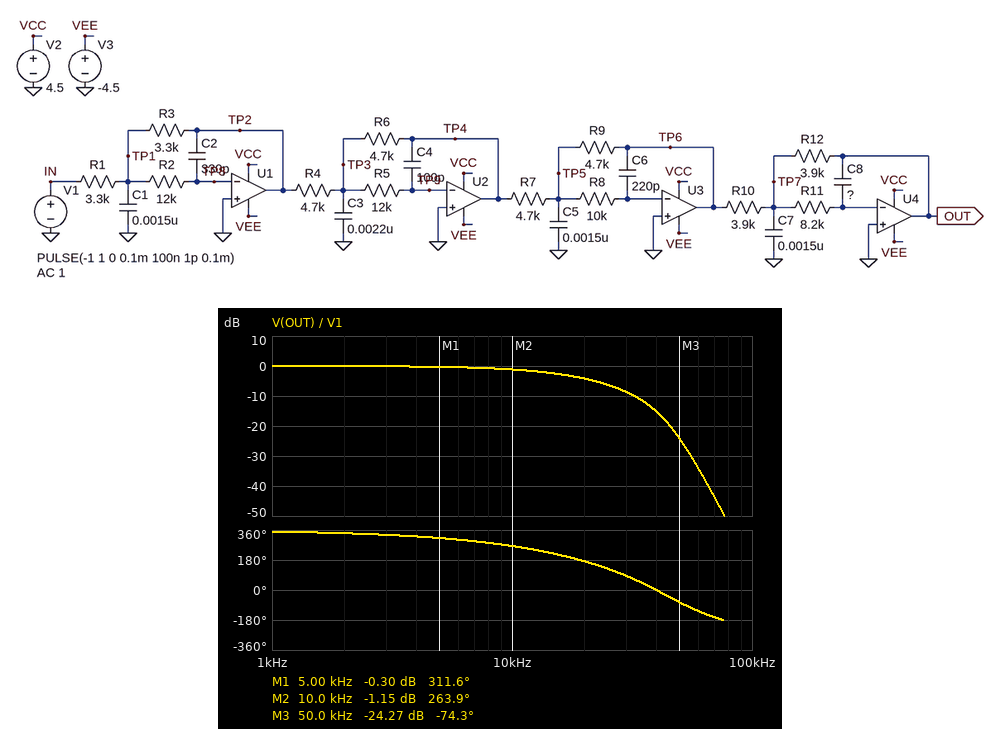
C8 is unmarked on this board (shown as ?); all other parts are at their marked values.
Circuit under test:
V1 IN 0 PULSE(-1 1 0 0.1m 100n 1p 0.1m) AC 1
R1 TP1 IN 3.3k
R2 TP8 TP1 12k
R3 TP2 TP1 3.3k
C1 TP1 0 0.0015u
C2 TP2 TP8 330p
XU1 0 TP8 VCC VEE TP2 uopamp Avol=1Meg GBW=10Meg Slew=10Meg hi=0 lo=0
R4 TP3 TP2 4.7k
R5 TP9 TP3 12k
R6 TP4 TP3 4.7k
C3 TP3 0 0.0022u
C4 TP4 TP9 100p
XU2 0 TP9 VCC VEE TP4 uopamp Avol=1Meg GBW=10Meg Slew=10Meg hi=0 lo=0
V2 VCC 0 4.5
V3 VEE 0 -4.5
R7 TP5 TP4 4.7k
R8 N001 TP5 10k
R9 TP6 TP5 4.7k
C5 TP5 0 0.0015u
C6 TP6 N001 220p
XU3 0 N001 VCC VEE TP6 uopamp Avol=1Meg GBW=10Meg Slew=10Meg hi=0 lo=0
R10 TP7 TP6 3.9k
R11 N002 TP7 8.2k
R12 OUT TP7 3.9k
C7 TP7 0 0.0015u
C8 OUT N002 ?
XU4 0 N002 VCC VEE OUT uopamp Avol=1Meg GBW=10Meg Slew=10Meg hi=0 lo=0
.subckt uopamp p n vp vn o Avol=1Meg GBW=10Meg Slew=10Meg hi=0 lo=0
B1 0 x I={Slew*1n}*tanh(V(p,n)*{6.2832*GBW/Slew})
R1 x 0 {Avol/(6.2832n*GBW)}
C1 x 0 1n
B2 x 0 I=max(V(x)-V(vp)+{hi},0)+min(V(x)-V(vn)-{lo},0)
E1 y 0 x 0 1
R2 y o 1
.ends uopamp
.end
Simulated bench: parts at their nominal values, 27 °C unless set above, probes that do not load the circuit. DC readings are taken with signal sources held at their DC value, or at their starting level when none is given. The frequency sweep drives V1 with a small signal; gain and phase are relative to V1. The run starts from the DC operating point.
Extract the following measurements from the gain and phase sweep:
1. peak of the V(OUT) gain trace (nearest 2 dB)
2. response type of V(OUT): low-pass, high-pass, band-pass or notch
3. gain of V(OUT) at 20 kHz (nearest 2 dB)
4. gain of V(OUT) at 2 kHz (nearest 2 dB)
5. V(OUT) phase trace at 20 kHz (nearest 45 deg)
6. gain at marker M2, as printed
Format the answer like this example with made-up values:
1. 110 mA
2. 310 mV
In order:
1. 0 dB
2. low-pass
3. -4 dB
4. 0 dB
5. 180 deg
6. -1.15 dB
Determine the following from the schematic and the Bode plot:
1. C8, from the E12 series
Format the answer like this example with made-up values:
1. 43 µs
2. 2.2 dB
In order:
1. 470 pF
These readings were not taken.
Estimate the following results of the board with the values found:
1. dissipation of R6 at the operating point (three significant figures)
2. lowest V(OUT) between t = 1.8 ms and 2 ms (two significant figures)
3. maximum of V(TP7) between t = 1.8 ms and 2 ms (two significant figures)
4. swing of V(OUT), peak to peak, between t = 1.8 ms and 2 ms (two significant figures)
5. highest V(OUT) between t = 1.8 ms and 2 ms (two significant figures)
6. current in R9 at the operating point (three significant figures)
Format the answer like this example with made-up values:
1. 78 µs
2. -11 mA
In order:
1. 213 µW
2. -620 mV
3. 320 mV
4. 1.3 V
5. 670 mV
6. 213 µA
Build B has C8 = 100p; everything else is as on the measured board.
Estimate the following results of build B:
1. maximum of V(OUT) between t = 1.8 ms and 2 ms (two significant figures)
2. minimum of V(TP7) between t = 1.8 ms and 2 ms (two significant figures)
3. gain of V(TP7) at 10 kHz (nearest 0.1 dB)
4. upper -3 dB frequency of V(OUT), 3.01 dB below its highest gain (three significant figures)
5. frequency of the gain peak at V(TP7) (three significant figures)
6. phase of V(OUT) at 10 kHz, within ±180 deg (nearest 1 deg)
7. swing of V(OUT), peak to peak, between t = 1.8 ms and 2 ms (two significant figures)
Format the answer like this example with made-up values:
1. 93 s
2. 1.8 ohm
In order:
1. 770 mV
2. -30 mV
3. -25.9 dB
4. 31.2 kHz
5. 32.2 kHz
6. -70 deg
7. 1.6 V
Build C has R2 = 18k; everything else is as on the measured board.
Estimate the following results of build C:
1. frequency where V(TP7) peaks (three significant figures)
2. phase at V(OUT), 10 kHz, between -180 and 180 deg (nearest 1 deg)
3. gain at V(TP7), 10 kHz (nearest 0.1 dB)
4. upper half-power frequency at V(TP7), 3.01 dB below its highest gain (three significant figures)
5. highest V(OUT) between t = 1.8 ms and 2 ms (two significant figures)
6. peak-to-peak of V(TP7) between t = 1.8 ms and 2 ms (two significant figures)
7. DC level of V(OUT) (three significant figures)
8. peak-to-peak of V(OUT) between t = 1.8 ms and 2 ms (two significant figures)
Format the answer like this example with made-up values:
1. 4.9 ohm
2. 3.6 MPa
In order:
1. 18.4 kHz
2. -107 deg
3. -14.3 dB
4. 33.5 kHz
5. 610 mV
6. 330 mV
7. -1.00 V
8. 1.1 V
